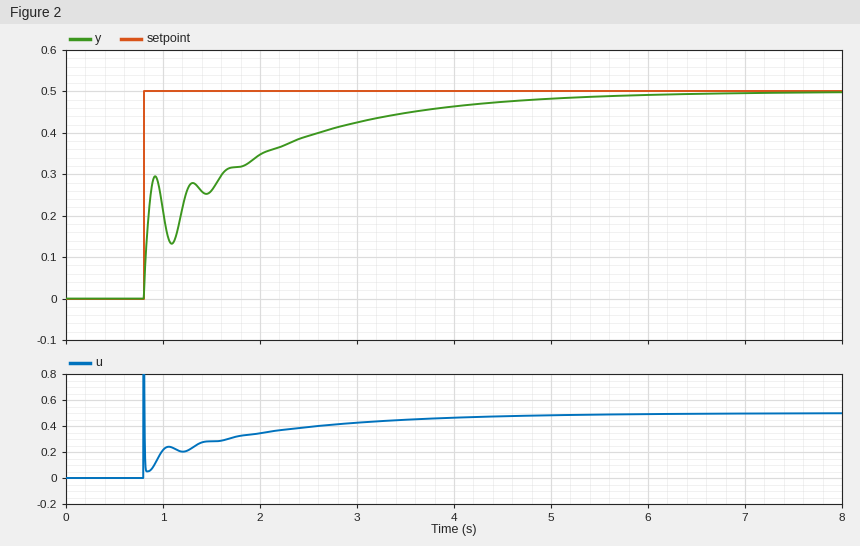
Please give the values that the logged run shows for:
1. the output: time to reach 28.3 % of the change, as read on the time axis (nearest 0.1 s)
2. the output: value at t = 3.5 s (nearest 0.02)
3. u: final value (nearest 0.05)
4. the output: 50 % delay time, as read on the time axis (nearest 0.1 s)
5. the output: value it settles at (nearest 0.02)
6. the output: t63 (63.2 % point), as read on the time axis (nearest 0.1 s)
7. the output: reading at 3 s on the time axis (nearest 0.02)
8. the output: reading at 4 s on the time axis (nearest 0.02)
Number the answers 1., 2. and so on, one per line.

1. 0.8 s
2. 0.44
3. 0.50
4. 0.9 s
5. 0.50
6. 1.7 s
7. 0.42
8. 0.46
